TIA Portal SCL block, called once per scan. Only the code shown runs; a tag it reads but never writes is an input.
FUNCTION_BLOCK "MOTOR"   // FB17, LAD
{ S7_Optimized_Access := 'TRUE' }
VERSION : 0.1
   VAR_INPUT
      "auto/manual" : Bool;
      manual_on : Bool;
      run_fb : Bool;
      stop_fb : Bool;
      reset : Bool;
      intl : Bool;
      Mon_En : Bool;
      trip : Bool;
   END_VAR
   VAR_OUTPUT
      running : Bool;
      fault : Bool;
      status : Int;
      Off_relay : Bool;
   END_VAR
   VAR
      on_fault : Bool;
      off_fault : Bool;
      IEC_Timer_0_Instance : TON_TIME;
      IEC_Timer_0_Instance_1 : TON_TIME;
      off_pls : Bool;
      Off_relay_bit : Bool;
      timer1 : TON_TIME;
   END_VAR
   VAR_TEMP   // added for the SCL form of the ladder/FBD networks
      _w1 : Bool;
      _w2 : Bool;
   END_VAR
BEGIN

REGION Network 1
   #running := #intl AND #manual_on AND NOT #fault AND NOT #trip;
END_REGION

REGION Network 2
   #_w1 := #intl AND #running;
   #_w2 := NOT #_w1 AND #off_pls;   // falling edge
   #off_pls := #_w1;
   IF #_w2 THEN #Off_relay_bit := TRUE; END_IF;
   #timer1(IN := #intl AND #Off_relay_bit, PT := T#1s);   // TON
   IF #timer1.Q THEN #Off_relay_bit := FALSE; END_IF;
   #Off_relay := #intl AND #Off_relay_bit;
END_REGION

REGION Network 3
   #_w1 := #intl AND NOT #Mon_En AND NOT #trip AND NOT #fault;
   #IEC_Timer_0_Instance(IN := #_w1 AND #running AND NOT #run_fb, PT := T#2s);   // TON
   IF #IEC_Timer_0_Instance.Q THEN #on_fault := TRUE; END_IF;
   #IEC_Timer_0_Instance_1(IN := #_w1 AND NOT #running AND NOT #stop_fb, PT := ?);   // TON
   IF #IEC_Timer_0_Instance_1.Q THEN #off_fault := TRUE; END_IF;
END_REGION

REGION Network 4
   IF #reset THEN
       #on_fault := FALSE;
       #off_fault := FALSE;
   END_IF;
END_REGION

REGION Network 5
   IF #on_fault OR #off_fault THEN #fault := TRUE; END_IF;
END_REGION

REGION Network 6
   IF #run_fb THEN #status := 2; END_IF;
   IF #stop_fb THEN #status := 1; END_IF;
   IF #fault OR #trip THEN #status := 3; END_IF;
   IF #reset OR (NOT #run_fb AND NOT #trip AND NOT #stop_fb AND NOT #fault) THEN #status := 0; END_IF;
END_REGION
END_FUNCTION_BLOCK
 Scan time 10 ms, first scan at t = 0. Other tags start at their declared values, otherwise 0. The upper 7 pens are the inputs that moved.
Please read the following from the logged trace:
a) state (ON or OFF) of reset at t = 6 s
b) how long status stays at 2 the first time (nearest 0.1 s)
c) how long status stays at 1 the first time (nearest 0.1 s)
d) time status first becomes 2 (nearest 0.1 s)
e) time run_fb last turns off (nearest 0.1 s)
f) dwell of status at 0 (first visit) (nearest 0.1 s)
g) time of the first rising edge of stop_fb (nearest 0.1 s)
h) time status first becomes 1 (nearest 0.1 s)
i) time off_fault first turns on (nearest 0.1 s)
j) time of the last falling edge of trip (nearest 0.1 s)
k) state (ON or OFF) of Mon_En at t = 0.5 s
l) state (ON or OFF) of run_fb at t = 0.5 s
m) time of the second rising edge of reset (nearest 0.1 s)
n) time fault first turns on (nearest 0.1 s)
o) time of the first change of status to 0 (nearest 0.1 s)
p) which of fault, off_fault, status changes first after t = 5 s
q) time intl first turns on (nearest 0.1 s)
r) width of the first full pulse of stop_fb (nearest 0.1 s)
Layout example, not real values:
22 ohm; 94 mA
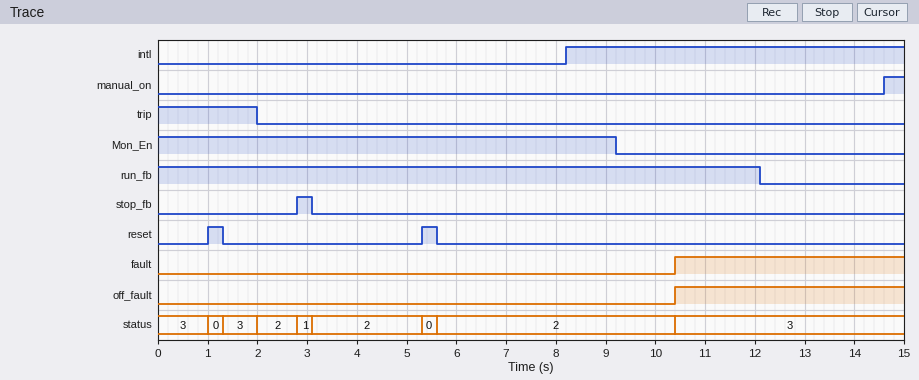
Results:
OFF; 0.8 s; 0.3 s; 2.0 s; 12.1 s; 0.3 s; 2.8 s; 2.8 s; 10.4 s; 2.0 s; ON; ON; 5.3 s; 10.4 s; 1.0 s; status; 8.2 s; 0.3 s
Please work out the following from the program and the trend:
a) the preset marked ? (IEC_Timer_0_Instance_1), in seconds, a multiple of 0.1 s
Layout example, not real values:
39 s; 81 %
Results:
1.2 s
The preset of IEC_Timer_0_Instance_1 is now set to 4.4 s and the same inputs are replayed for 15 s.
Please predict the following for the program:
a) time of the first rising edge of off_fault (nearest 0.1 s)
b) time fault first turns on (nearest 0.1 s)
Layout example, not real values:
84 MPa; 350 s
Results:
13.6 s; 13.6 s
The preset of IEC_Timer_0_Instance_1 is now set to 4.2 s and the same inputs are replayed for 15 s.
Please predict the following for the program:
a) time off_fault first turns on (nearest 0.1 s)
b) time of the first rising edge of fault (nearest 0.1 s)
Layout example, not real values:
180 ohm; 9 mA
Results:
13.4 s; 13.4 s
